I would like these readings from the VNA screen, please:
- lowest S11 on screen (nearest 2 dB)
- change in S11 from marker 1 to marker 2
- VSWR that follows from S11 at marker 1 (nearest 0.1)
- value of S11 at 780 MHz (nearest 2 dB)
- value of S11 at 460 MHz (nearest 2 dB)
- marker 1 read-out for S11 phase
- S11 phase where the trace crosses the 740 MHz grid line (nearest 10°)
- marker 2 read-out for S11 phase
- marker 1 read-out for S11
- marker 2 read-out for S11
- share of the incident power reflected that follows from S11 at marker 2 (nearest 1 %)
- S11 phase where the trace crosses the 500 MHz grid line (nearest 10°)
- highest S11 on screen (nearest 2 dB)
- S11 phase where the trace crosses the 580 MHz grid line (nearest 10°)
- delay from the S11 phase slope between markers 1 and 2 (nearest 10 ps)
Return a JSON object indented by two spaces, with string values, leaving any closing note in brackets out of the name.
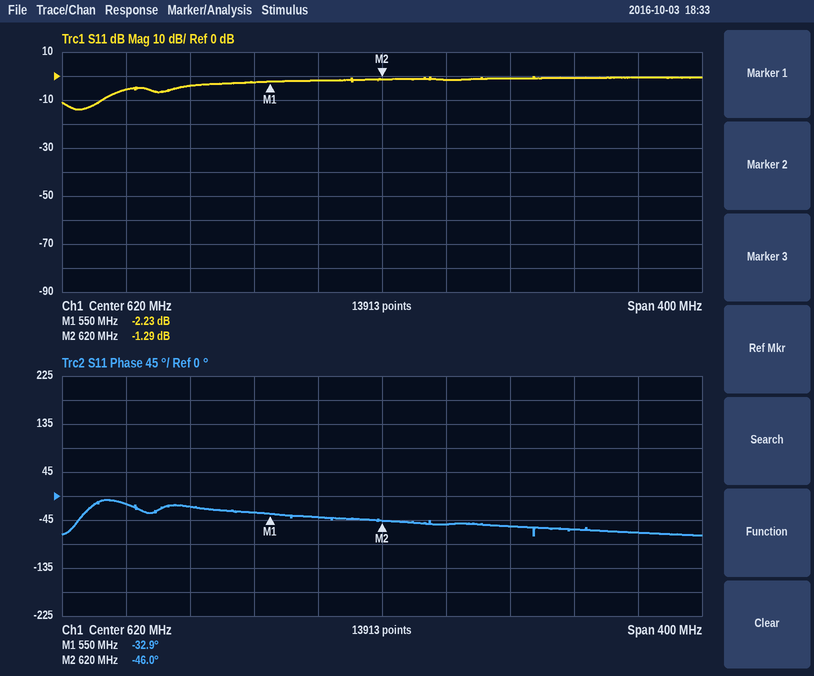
{
  "lowest S11 on screen": "-14 dB",
  "change in S11 from marker 1 to marker 2": "0.94 dB",
  "VSWR that follows from S11 at marker 1": "7.8",
  "value of S11 at 780 MHz": "0 dB",
  "value of S11 at 460 MHz": "-6 dB",
  "marker 1 read-out for S11 phase": "-32.9°",
  "S11 phase where the trace crosses the 740 MHz grid line": "-60°",
  "marker 2 read-out for S11 phase": "-46.0°",
  "marker 1 read-out for S11": "-2.23 dB",
  "marker 2 read-out for S11": "-1.29 dB",
  "share of the incident power reflected that follows from S11 at marker 2": "74 %",
  "S11 phase where the trace crosses the 500 MHz grid line": "-20°",
  "highest S11 on screen": "0 dB",
  "S11 phase where the trace crosses the 580 MHz grid line": "-40°",
  "delay from the S11 phase slope between markers 1 and 2": "520 ps"
}
